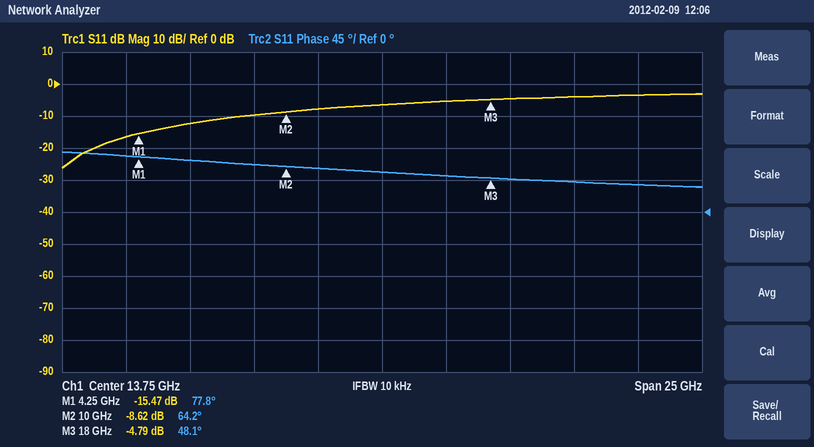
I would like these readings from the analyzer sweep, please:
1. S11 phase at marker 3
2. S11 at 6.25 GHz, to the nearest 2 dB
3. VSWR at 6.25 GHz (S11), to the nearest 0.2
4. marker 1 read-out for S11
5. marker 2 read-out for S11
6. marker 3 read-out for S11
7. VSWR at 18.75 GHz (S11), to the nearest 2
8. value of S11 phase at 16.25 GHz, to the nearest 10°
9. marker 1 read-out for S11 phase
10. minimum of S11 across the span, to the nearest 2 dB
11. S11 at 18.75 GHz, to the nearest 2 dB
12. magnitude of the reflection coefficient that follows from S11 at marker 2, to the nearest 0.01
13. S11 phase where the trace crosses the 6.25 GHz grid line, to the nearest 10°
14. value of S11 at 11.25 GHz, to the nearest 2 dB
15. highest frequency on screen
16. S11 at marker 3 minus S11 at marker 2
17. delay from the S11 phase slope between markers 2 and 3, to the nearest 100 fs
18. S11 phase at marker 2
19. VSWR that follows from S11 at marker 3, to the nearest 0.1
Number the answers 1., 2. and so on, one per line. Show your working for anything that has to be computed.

1. 48.1°
2. -12 dB
3. |Γ| = 10^(-12/20) = 0.2512; VSWR = (1 + 0.2512)/(1 − 0.2512) ≈ 1.67, so 1.6 to the nearest 0.2
4. -15.47 dB
5. -8.62 dB
6. -4.79 dB
7. |Γ| = 10^(-4/20) = 0.6310; VSWR = (1 + 0.6310)/(1 − 0.6310) ≈ 4
8. 50°
9. 77.8°
10. -26 dB
11. -4 dB
12. 10^(-8.62/20) ≈ 0.37
13. 70°
14. -8 dB
15. 26.25 GHz
16. -4.79 − (-8.62) = 3.83 dB
17. −(48.1° − (64.2°))/(360° × 8 GHz) ≈ 5.6 ps
18. 64.2°
19. (1 + 0.5761)/(1 − 0.5761) ≈ 3.7
